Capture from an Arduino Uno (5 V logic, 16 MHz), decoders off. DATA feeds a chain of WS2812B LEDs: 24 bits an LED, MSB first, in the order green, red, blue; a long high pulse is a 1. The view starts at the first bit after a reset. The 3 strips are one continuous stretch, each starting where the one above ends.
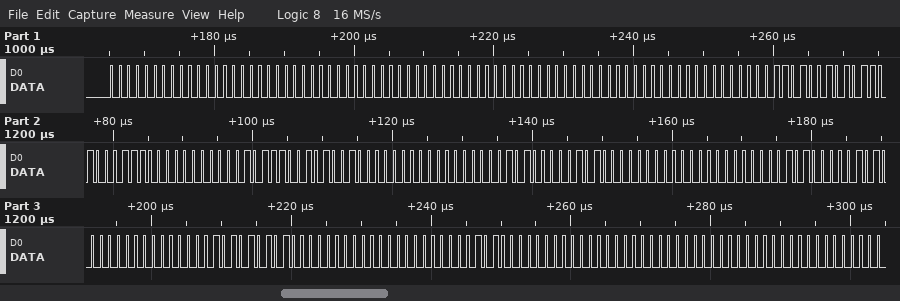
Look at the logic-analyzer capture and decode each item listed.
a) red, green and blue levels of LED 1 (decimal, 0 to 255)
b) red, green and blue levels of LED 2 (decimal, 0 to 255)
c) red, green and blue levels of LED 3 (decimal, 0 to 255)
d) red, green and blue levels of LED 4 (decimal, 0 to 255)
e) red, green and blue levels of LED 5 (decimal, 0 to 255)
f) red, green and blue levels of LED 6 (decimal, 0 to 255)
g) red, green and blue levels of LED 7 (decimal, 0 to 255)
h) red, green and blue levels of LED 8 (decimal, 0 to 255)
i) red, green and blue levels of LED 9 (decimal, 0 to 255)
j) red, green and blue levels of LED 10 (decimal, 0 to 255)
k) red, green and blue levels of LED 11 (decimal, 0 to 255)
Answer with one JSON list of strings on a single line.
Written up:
["0, 0, 0", "0, 0, 0", "0, 0, 0", "43, 13, 71", "23, 0, 41", "0, 0, 80", "0, 80, 0", "80, 80, 0", "80, 21, 0", "80, 0, 0", "0, 0, 0"]
